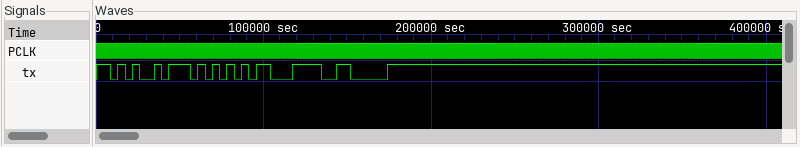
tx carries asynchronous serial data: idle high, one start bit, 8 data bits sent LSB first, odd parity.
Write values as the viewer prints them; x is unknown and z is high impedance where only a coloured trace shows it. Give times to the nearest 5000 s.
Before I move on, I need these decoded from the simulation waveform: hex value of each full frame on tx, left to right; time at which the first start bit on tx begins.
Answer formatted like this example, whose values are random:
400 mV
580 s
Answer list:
A5, 55, 3C, F0
10000 s
